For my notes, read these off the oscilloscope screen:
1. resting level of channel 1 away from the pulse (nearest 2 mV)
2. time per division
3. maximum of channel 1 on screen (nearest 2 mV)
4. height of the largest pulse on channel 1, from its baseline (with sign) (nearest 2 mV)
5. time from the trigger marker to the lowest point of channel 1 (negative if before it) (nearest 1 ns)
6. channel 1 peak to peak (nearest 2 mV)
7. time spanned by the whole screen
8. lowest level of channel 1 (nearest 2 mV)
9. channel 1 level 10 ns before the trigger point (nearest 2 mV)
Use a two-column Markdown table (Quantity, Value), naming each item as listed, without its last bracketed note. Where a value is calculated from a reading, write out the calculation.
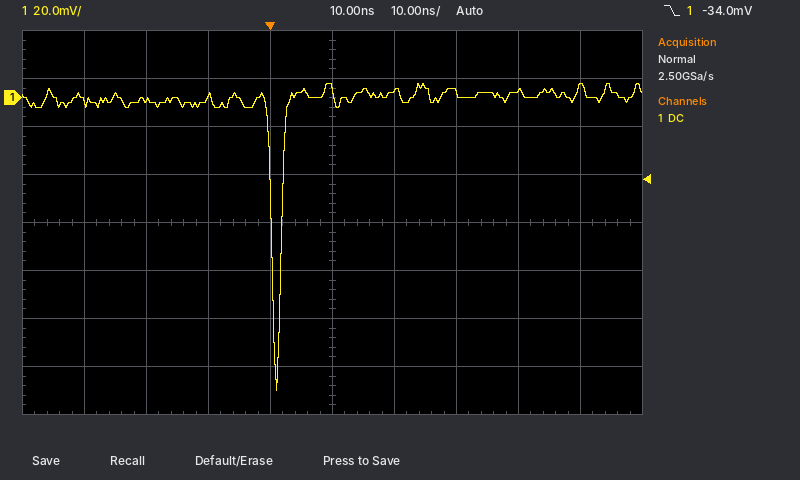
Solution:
| Quantity | Value |
|---|---|
| resting level of channel 1 away from the pulse | 0 mV |
| time per division | 10 ns |
| maximum of channel 1 on screen | 6 mV |
| height of the largest pulse on channel 1, from its baseline (with sign) | -122 mV − (0 mV) = -122 mV |
| time from the trigger marker to the lowest point of channel 1 (negative if before it) | +1 ns |
| channel 1 peak to peak | 6 mV − (-122 mV) = 128 mV |
| time spanned by the whole screen | 100 ns |
| lowest level of channel 1 | -122 mV |
| channel 1 level 10 ns before the trigger point | 0 mV |
